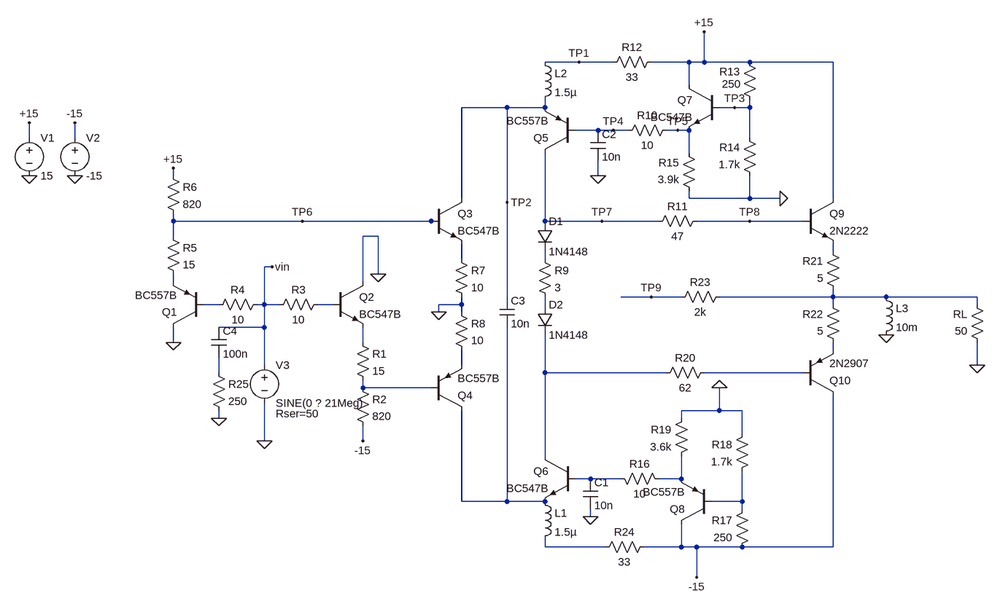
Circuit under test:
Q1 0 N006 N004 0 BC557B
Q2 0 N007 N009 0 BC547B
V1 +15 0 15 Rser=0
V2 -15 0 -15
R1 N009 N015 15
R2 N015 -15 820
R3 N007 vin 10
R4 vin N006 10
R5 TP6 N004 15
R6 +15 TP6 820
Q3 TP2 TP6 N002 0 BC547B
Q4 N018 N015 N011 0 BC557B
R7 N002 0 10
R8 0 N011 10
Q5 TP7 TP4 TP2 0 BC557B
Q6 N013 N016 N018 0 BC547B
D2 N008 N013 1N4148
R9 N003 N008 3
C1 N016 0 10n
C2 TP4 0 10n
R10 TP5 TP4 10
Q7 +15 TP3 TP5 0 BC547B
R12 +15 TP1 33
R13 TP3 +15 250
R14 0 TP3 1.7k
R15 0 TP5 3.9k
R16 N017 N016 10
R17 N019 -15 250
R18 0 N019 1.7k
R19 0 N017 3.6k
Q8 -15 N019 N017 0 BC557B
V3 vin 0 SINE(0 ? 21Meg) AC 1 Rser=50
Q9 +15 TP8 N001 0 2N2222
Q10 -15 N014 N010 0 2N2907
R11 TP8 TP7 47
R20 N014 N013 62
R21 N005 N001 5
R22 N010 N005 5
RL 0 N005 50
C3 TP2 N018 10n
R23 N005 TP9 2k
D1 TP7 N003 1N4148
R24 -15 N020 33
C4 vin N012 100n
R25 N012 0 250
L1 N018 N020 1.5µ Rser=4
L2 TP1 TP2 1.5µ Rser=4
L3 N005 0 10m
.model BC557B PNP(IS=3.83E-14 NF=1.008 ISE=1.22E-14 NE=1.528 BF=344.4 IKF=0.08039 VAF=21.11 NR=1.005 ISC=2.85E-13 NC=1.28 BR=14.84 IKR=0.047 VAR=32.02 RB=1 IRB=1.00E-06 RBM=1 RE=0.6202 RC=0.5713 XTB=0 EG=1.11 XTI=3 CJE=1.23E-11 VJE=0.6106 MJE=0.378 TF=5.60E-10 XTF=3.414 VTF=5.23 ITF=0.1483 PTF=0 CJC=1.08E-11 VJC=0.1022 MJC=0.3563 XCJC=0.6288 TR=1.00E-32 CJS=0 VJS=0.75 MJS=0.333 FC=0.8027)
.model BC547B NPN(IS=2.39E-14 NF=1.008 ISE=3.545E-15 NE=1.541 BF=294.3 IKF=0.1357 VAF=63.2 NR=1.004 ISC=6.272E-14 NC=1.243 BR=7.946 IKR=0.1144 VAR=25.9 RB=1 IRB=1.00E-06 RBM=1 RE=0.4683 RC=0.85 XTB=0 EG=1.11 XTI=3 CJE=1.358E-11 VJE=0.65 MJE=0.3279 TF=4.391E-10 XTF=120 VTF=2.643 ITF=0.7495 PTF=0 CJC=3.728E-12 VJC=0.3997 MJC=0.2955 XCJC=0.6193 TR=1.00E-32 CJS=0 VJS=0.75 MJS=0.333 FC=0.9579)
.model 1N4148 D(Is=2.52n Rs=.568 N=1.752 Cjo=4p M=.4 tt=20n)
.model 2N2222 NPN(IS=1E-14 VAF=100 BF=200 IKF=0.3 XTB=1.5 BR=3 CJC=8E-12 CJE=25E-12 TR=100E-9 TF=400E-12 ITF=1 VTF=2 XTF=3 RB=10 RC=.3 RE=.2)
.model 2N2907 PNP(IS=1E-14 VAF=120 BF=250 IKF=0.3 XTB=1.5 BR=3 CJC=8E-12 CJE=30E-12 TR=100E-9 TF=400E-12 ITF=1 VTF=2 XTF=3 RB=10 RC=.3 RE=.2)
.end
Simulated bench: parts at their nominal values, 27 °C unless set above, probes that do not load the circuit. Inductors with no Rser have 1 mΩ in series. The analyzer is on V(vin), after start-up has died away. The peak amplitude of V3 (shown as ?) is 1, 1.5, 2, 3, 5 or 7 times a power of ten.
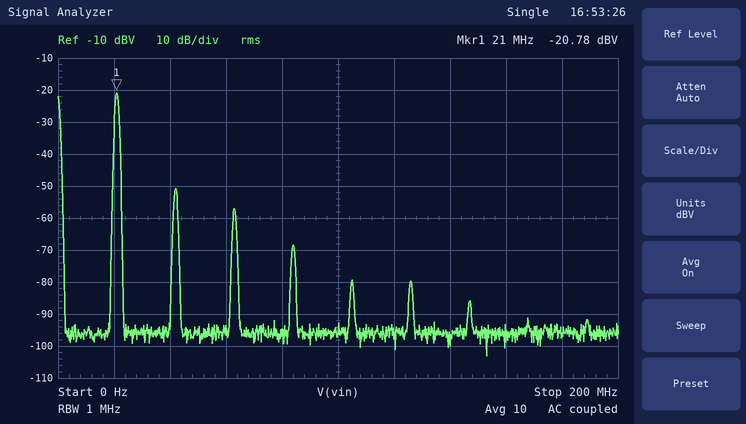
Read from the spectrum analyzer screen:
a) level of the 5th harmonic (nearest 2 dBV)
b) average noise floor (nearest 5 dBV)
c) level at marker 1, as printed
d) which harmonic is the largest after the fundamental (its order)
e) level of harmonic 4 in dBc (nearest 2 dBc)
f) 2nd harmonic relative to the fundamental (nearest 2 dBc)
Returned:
-80 dBV
-95 dBV
-20.78 dBV
2
-48 dBc
-30 dBc
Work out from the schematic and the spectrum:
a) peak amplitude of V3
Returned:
150 mV
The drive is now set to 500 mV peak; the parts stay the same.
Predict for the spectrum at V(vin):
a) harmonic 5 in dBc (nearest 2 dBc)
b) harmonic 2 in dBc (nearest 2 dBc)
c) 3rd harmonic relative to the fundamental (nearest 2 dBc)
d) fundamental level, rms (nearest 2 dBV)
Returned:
-38 dBc
-18 dBc
-28 dBc
-10 dBV
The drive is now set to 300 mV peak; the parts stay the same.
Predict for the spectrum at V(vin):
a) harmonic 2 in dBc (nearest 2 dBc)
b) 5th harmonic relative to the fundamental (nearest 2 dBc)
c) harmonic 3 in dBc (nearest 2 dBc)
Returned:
-22 dBc
-42 dBc
-30 dBc
